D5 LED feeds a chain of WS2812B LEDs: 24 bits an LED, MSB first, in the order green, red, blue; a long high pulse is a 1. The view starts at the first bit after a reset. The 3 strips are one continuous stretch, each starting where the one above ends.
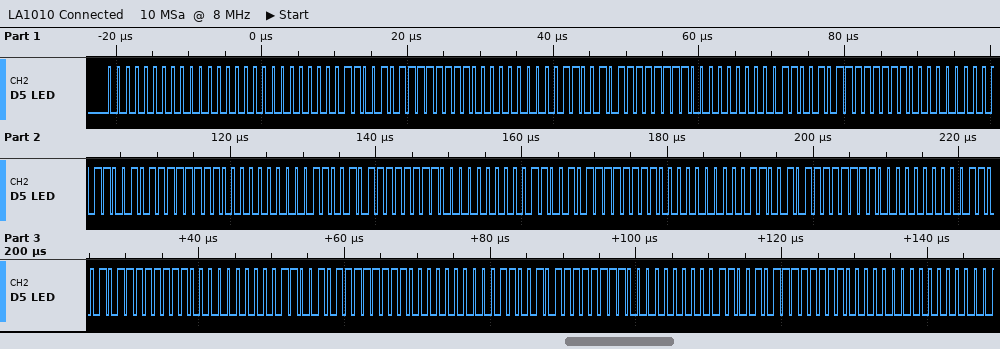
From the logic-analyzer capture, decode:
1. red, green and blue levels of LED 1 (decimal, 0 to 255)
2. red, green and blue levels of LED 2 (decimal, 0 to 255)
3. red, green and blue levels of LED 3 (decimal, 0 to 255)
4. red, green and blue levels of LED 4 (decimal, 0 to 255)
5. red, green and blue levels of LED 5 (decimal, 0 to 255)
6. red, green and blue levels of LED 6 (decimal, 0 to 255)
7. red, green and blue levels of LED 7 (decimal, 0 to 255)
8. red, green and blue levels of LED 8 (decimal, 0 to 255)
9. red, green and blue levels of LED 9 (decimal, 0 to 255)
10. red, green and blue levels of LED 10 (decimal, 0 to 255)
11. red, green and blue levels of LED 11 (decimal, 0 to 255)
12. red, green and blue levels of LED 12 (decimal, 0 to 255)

0, 0, 0
255, 50, 0
255, 50, 0
255, 50, 0
255, 50, 0
255, 50, 0
255, 50, 0
255, 50, 0
255, 50, 0
255, 50, 0
255, 50, 0
255, 50, 0
